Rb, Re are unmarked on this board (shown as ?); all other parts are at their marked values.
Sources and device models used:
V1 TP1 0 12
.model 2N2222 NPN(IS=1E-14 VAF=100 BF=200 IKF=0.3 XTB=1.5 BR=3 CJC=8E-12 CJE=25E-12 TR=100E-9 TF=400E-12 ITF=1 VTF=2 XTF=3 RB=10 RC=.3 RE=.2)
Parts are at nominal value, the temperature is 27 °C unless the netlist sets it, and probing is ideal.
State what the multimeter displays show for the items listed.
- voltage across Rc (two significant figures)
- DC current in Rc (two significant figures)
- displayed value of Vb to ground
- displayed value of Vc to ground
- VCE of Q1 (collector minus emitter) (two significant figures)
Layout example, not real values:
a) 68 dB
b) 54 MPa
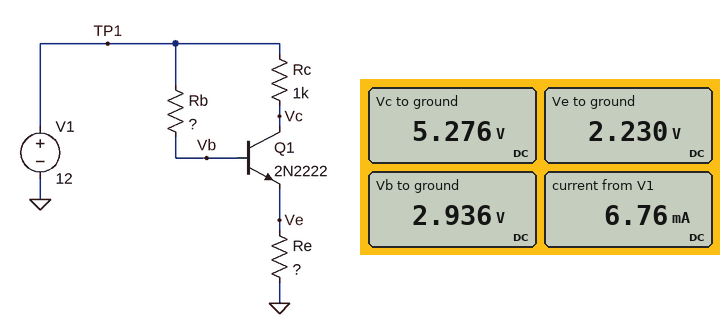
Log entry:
a) 6.7 V
b) 6.7 mA
c) 2.936 V
d) 5.276 V
e) 3.0 V
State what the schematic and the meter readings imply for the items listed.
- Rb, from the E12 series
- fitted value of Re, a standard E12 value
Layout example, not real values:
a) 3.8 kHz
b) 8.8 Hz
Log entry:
a) 270 kΩ
b) 330 Ω
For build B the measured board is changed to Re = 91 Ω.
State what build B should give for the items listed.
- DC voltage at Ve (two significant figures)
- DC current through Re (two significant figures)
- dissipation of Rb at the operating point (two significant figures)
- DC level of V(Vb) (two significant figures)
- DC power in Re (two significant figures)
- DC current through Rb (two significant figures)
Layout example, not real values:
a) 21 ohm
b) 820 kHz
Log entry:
a) 720 mV
b) 7.9 mA
c) 410 µW
d) 1.4 V
e) 5.7 mW
f) 39 µA
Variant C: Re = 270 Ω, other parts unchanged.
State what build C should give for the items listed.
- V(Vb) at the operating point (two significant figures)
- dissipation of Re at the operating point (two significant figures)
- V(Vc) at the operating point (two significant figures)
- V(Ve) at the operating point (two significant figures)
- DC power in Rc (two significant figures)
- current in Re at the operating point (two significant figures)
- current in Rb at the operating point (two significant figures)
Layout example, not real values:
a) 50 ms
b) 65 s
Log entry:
a) 2.6 V
b) 13 mW
c) 5.0 V
d) 1.9 V
e) 49 mW
f) 7.0 mA
g) 35 µA
